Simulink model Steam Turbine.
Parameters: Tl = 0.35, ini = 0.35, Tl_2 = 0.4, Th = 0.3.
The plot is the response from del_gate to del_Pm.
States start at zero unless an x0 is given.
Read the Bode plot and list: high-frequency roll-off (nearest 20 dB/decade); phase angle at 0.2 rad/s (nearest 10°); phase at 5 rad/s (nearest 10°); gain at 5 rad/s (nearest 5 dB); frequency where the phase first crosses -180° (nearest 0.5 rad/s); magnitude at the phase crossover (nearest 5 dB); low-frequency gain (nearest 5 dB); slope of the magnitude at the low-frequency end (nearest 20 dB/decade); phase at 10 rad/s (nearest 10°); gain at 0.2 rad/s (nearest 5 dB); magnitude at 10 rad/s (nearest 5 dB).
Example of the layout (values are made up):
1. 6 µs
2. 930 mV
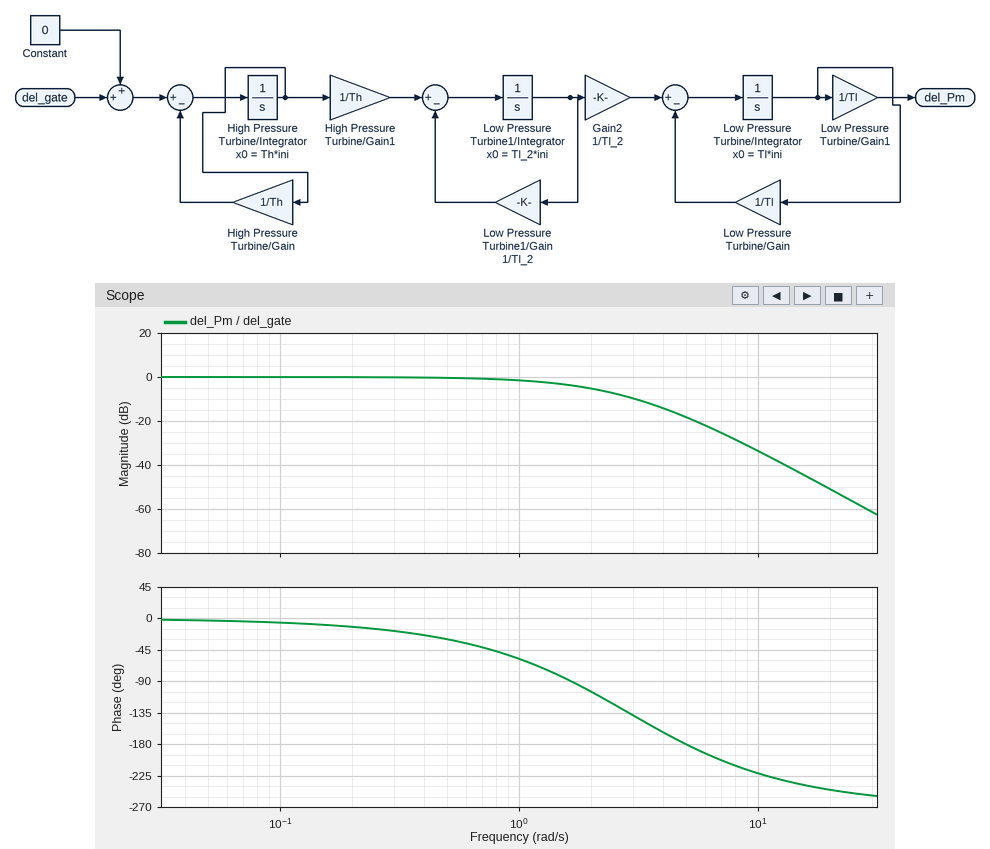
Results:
1. -60 dB/decade
2. -10°
3. -180°
4. -20 dB
5. 5.0 rad/s
6. -20 dB
7. 0 dB
8. 0 dB/decade
9. -220°
10. 0 dB
11. -35 dB
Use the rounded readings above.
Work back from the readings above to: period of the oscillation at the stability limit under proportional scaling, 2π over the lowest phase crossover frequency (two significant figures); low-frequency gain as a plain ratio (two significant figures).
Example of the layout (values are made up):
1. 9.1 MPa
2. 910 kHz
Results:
1. 1.3 s
2. 1.0
